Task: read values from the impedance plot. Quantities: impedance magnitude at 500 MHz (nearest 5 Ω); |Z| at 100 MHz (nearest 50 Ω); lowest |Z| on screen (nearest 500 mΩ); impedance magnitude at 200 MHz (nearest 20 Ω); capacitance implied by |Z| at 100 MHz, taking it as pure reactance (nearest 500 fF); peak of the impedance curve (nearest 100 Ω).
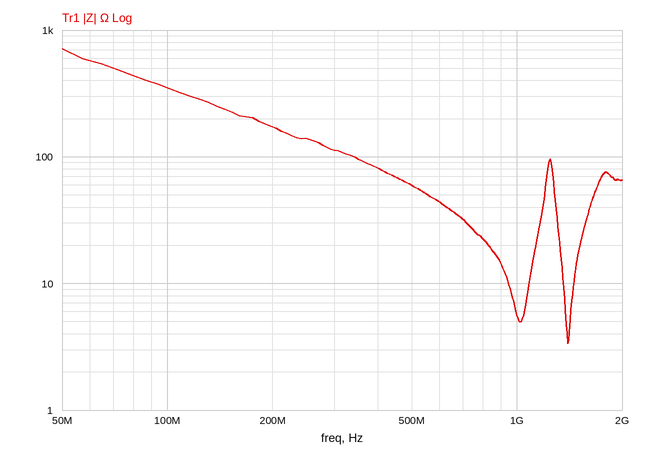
60 Ω
350 Ω
3.5 Ω
180 Ω
4.5 pF
700 Ω
